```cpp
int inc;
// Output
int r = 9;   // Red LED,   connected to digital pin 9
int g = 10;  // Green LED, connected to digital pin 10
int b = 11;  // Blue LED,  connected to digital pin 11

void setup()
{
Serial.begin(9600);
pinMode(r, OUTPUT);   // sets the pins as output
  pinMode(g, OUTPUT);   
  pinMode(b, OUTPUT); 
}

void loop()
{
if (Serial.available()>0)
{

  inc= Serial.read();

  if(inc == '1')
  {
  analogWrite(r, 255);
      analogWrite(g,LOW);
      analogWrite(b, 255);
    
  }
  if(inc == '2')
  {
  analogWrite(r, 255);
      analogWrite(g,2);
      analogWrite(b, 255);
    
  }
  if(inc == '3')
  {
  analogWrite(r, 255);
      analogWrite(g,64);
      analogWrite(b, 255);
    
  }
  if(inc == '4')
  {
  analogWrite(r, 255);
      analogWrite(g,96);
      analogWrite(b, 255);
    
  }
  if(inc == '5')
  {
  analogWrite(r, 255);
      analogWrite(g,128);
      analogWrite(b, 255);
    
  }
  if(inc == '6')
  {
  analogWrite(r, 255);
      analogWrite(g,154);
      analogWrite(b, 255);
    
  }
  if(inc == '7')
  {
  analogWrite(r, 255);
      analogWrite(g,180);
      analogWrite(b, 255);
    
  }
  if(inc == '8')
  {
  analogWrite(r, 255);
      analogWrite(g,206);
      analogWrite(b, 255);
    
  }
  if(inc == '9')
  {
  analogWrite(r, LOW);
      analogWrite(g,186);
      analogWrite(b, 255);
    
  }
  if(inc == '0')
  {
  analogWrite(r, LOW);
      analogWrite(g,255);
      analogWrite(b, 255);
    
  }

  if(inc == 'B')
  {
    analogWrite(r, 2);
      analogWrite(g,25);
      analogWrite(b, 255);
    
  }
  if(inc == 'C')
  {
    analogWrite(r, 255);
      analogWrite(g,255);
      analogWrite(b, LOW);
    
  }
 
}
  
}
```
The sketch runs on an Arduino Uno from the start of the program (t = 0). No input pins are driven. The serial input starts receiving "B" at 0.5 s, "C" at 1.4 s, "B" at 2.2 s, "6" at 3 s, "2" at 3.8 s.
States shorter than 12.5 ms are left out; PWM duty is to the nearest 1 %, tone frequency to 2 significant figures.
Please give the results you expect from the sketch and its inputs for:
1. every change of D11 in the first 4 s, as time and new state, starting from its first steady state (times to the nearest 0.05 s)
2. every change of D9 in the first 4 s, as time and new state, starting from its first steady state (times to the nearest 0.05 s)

0 s low; 0.5 s high; 1.4 s low; 2.2 s high
0 s low; 0.5 s PWM 1 %; 1.4 s high; 2.2 s PWM 1 %; 3 s high
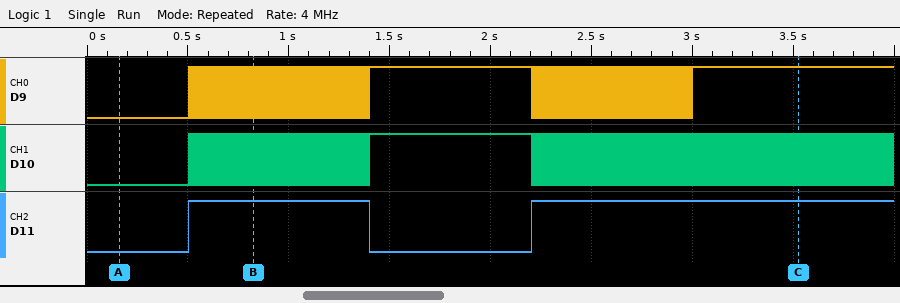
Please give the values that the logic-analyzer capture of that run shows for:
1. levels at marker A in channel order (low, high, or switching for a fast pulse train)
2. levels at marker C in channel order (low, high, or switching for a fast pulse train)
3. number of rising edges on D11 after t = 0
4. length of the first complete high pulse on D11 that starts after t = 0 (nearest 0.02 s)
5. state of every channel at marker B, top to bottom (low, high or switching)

D9 low, D10 low, D11 low
D9 high, D10 switching, D11 high
2
0.90 s
D9 switching, D10 switching, D11 high
